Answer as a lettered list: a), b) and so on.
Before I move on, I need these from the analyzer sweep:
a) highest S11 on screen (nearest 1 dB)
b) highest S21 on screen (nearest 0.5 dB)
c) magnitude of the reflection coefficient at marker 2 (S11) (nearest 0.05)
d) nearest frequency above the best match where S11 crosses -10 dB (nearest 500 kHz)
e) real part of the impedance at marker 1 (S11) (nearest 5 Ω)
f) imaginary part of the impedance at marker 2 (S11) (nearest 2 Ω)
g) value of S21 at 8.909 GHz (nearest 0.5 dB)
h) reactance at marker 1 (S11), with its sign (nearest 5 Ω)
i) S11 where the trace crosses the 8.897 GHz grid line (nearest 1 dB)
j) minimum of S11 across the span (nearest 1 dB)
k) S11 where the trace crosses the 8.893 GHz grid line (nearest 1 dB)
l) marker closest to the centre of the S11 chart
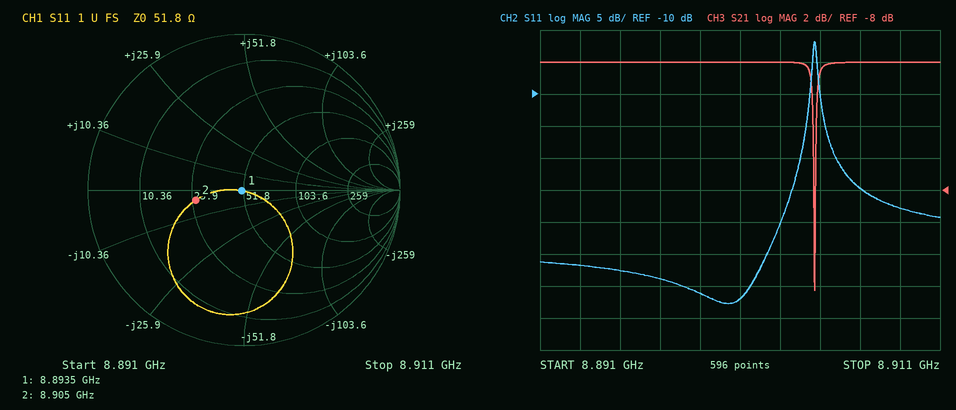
a) -2 dB
b) 0.0 dB
c) 0.30
d) 8.9045 GHz
e) 50 Ω
f) -4 Ω
g) 0.0 dB
h) 0 Ω
i) -39 dB
j) -43 dB
k) -37 dB
l) marker 1
